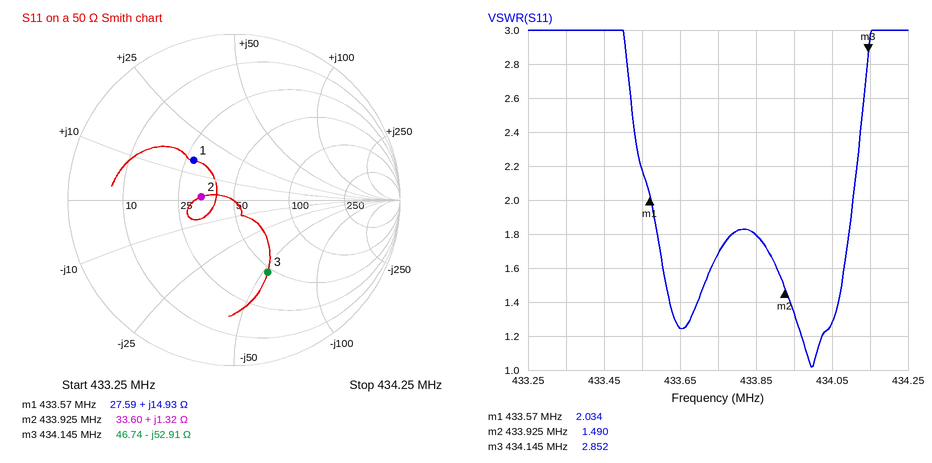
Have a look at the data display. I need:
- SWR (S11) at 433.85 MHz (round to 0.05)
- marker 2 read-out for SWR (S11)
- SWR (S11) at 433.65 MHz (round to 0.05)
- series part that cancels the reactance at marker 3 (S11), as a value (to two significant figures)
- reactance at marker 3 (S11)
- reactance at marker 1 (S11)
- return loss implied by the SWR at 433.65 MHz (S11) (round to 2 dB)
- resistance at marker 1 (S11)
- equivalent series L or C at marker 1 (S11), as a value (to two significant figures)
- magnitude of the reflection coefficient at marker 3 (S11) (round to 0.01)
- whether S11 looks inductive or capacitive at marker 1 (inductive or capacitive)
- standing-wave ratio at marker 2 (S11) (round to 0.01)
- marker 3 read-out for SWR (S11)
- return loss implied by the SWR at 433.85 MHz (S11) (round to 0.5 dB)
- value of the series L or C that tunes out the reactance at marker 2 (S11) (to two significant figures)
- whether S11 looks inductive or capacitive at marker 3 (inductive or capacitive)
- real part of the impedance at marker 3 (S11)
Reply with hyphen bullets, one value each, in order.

- 1.80
- 1.490
- 1.25
- 19 nH
- -52.91 Ω
- +14.93 Ω
- 20 dB
- 27.59 Ω
- 5.5 nH
- 0.48
- inductive
- 1.49
- 2.852
- 11.0 dB
- 280 pF
- capacitive
- 46.74 Ω
